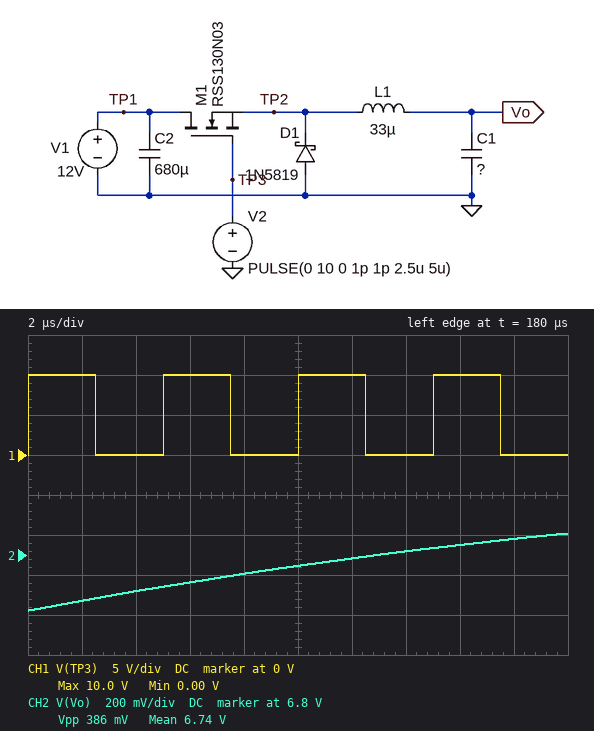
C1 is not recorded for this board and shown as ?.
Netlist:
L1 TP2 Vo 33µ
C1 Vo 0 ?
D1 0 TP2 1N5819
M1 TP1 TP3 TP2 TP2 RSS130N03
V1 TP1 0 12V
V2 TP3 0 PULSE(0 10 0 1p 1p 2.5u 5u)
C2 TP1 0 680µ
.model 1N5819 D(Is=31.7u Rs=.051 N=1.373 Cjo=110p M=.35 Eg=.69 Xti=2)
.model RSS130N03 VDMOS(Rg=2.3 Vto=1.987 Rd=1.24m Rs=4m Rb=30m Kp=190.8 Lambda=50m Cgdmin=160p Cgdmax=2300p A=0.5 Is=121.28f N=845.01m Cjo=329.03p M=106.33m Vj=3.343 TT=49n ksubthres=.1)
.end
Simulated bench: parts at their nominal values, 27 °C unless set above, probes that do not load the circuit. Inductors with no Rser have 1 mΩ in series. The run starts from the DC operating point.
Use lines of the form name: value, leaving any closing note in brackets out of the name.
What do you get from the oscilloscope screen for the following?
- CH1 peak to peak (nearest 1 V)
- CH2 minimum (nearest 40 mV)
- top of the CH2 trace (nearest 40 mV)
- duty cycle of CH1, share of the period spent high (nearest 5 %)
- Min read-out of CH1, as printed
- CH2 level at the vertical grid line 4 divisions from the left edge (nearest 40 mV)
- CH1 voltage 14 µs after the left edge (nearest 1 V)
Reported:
CH1 peak to peak: 10 V
CH2 minimum: 6.52 V
top of the CH2 trace: 6.92 V
duty cycle of CH1, share of the period spent high: 50 %
Min read-out of CH1, as printed: 0.00 V
CH2 level at the vertical grid line 4 divisions from the left edge: 6.72 V
CH1 voltage 14 µs after the left edge: 0 V
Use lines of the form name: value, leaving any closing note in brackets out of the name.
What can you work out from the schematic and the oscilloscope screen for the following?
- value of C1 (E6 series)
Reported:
value of C1: 150 µF
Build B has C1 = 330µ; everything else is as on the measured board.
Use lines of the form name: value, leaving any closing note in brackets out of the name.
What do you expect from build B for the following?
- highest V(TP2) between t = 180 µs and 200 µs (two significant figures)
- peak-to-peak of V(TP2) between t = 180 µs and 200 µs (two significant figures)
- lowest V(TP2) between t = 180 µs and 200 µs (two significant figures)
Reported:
highest V(TP2) between t = 180 µs and 200 µs: 7.7 V
peak-to-peak of V(TP2) between t = 180 µs and 200 µs: 8.7 V
lowest V(TP2) between t = 180 µs and 200 µs: -1.0 V
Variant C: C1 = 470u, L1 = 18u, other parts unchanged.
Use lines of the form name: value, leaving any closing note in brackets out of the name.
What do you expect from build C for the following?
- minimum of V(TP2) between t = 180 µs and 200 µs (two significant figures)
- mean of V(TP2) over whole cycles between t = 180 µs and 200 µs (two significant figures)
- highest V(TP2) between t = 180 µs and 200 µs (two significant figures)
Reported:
minimum of V(TP2) between t = 180 µs and 200 µs: -1.2 V
mean of V(TP2) over whole cycles between t = 180 µs and 200 µs: 3.2 V
highest V(TP2) between t = 180 µs and 200 µs: 7.6 V
